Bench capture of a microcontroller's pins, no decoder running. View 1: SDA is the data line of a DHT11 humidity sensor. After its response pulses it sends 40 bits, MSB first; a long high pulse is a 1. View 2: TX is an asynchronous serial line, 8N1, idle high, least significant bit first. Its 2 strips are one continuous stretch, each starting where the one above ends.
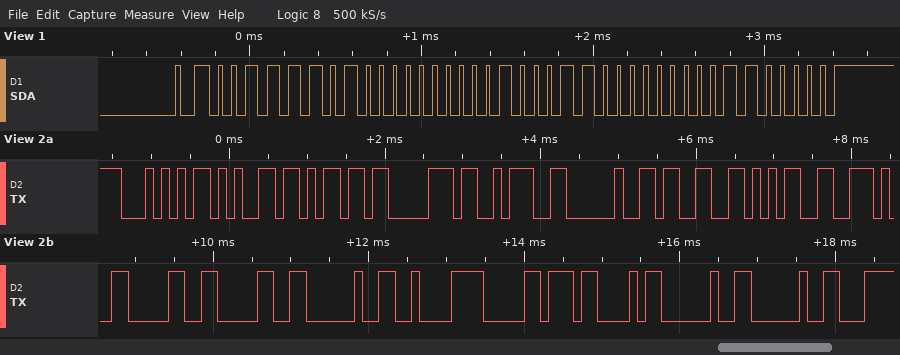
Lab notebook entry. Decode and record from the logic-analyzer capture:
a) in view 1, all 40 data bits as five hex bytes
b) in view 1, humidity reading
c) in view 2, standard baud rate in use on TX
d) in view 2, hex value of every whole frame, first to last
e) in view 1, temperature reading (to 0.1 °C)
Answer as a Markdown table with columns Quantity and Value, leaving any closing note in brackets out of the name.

| Quantity | Value |
|---|---|
| in view 1, all 40 data bits as five hex bytes | 3D 00 23 00 60 |
| in view 1, humidity reading | 61 % |
| in view 2, standard baud rate in use on TX | 9600 baud |
| in view 2, hex value of every whole frame, first to last | 0x54 0x65 0x6D 0x70 0x3A 0x20 0x33 0x35 0x2E 0x30 0x30 0x20 0xC2 0xB0 0x43 0x20 0x20 |
| in view 1, temperature reading | 35.0 °C |
